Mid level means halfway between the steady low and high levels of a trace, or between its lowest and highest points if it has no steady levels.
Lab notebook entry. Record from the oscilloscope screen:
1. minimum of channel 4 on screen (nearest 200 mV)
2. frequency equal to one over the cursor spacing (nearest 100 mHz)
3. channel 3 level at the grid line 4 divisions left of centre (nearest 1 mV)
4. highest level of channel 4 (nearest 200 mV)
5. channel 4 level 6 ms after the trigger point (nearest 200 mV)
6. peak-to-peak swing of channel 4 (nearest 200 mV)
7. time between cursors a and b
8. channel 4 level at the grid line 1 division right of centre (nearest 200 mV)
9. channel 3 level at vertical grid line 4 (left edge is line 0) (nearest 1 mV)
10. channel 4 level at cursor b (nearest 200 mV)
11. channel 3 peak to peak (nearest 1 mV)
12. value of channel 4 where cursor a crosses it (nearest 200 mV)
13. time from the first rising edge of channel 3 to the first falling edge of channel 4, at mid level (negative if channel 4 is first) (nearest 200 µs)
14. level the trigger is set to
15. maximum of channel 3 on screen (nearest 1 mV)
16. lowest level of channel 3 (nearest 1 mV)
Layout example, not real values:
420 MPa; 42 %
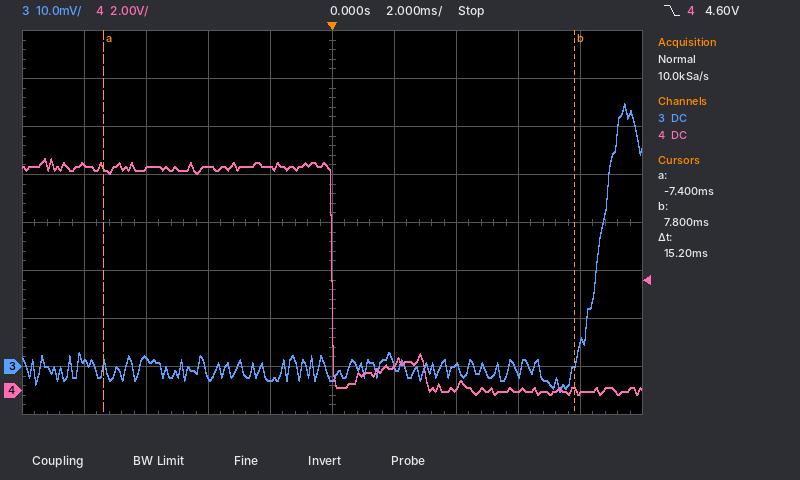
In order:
-200 mV; 65.8 Hz; 1 mV; 9.6 V; 0.0 V; 9.8 V; 15.2 ms; 1.0 V; -3 mV; 0.0 V; 60 mV; 9.4 V; -8.6 ms; 4.60 V; 55 mV; -5 mV
